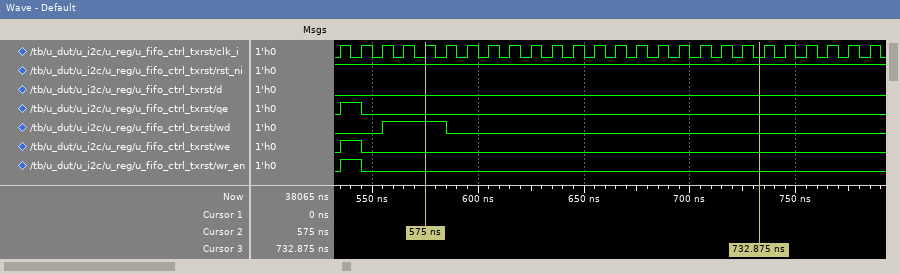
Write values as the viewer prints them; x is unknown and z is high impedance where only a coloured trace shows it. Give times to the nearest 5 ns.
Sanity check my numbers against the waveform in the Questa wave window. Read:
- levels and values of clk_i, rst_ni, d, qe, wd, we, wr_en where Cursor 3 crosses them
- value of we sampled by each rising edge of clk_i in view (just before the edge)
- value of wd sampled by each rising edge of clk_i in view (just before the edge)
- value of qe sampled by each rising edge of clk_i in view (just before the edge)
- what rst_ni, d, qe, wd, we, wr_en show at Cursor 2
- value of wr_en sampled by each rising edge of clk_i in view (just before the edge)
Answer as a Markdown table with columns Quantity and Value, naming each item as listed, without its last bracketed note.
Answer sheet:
| Quantity | Value |
|---|---|
| levels and values of clk_i, rst_ni, d, qe, wd, we, wr_en where Cursor 3 crosses them | clk_i=0, rst_ni=1, d=0, qe=0, wd=0, we=0, wr_en=0 |
| value of we sampled by each rising edge of clk_i in view | 0 1 0 0 0 0 0 0 0 0 0 0 0 0 0 0 0 0 0 0 0 0 0 0 0 0 |
| value of wd sampled by each rising edge of clk_i in view | 0 0 0 1 1 1 0 0 0 0 0 0 0 0 0 0 0 0 0 0 0 0 0 0 0 0 |
| value of qe sampled by each rising edge of clk_i in view | 0 1 0 0 0 0 0 0 0 0 0 0 0 0 0 0 0 0 0 0 0 0 0 0 0 0 |
| what rst_ni, d, qe, wd, we, wr_en show at Cursor 2 | rst_ni=1, d=0, qe=0, wd=1, we=0, wr_en=0 |
| value of wr_en sampled by each rising edge of clk_i in view | 0 1 0 0 0 0 0 0 0 0 0 0 0 0 0 0 0 0 0 0 0 0 0 0 0 0 |
